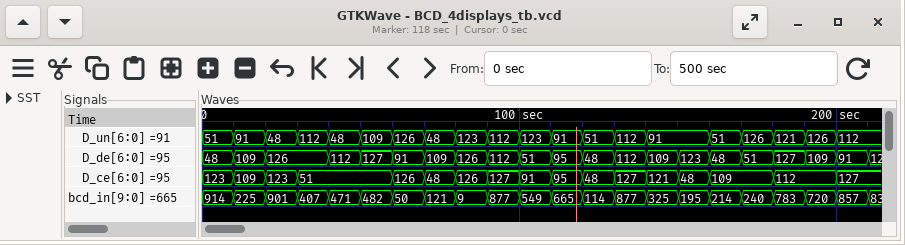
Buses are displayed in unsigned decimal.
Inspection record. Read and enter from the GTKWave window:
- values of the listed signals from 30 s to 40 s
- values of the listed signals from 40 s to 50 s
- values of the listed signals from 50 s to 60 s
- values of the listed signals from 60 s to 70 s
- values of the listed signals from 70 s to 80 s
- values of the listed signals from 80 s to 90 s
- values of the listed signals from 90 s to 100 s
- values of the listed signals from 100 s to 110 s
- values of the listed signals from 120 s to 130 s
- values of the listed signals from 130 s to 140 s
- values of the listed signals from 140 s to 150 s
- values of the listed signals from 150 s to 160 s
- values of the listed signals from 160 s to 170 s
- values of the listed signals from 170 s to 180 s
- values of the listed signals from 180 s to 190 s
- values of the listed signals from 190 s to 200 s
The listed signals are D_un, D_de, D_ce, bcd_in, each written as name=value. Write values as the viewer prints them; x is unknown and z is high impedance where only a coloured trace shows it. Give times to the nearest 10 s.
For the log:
D_un=112, D_de=126, D_ce=51, bcd_in=407
D_un=48, D_de=112, D_ce=51, bcd_in=471
D_un=109, D_de=127, D_ce=51, bcd_in=482
D_un=126, D_de=91, D_ce=126, bcd_in=50
D_un=48, D_de=109, D_ce=48, bcd_in=121
D_un=123, D_de=126, D_ce=126, bcd_in=9
D_un=112, D_de=112, D_ce=127, bcd_in=877
D_un=123, D_de=51, D_ce=91, bcd_in=549
D_un=51, D_de=48, D_ce=48, bcd_in=114
D_un=112, D_de=112, D_ce=127, bcd_in=877
D_un=91, D_de=109, D_ce=121, bcd_in=325
D_un=91, D_de=123, D_ce=48, bcd_in=195
D_un=51, D_de=48, D_ce=109, bcd_in=214
D_un=126, D_de=51, D_ce=109, bcd_in=240
D_un=121, D_de=127, D_ce=112, bcd_in=783
D_un=126, D_de=109, D_ce=112, bcd_in=720
